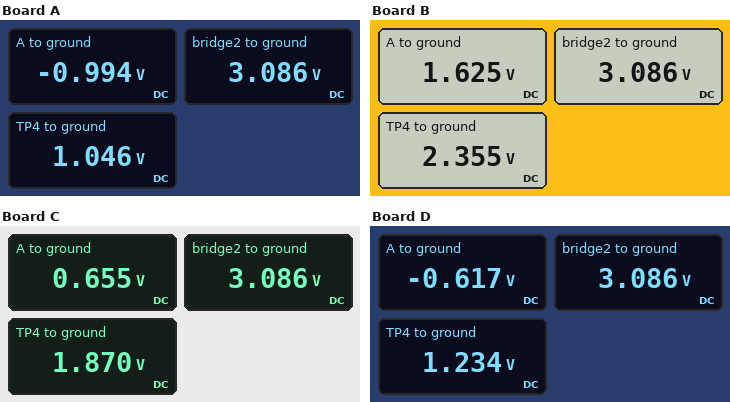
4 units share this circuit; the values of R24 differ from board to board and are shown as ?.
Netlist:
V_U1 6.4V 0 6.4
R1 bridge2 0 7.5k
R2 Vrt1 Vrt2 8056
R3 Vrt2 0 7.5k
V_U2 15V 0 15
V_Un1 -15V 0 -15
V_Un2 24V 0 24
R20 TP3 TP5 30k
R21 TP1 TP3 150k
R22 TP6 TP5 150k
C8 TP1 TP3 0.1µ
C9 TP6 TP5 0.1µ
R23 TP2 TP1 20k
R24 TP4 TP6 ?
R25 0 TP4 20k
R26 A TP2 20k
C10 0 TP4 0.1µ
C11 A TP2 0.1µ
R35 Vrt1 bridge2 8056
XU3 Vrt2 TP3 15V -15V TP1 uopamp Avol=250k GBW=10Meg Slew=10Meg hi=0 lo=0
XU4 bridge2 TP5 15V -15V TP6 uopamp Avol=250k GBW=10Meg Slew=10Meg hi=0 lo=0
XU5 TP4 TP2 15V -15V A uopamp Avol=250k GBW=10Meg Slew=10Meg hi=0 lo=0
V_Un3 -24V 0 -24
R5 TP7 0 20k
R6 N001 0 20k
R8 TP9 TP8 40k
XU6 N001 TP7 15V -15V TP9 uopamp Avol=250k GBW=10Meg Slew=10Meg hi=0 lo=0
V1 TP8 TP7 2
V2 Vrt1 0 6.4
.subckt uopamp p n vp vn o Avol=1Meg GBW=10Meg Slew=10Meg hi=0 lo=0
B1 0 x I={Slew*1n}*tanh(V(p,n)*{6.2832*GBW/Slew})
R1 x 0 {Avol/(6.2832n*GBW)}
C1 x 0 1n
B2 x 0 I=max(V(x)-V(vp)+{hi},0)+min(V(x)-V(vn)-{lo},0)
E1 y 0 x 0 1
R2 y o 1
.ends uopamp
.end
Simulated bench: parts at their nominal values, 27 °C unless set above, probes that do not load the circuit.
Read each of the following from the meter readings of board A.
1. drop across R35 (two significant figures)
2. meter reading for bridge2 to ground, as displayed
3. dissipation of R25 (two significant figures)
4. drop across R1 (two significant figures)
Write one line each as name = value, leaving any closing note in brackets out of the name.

drop across R35 = 3.3 V
meter reading for bridge2 to ground, as displayed = 3.086 V
dissipation of R25 = 55 µW
drop across R1 = 3.1 V
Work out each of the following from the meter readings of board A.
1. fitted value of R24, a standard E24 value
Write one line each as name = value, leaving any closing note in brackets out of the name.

fitted value of R24, a standard E24 value = 39 kΩ
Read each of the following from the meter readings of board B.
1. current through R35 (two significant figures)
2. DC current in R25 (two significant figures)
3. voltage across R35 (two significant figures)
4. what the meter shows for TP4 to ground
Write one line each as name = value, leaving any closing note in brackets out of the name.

current through R35 = 410 µA
DC current in R25 = 120 µA
voltage across R35 = 3.3 V
what the meter shows for TP4 to ground = 2.355 V
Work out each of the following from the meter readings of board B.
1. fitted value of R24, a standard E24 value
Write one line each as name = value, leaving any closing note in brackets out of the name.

fitted value of R24, a standard E24 value = 6.2 kΩ
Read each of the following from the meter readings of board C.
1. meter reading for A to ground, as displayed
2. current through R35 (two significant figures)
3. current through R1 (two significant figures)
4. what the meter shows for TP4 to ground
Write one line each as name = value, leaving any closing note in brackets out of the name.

meter reading for A to ground, as displayed = 0.655 V
current through R35 = 410 µA
current through R1 = 410 µA
what the meter shows for TP4 to ground = 1.870 V
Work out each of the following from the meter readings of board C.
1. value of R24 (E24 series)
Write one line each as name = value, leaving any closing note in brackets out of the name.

value of R24 = 13 kΩ
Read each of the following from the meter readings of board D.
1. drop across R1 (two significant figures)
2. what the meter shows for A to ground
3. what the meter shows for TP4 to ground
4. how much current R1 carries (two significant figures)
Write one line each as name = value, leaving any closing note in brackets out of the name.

drop across R1 = 3.1 V
what the meter shows for A to ground = -0.617 V
what the meter shows for TP4 to ground = 1.234 V
how much current R1 carries = 410 µA
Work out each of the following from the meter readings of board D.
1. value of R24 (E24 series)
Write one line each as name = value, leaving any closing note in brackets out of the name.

value of R24 = 30 kΩ
